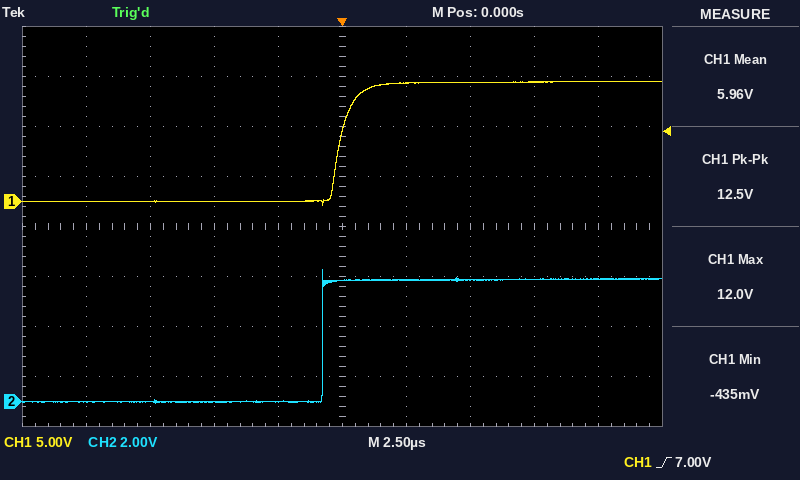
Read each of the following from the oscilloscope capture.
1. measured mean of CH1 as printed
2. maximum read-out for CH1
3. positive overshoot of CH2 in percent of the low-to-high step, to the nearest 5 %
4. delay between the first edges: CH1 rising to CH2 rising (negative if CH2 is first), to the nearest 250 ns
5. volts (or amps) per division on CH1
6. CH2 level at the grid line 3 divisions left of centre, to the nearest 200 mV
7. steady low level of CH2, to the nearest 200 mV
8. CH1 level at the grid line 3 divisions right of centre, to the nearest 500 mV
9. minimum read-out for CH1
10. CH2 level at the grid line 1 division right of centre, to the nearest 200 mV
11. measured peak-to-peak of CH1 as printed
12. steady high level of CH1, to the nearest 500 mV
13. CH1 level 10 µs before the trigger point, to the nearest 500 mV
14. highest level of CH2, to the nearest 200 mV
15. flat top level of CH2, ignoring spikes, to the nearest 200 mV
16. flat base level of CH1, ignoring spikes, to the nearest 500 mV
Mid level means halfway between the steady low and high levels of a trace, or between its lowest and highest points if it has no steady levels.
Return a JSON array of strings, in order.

["5.96 V", "12.0 V", "10 %", "-750 ns", "5 V", "0.0 V", "0.0 V", "12.0 V", "-435 mV", "4.8 V", "12.5 V", "12.0 V", "0.0 V", "5.2 V", "4.8 V", "0.0 V"]
